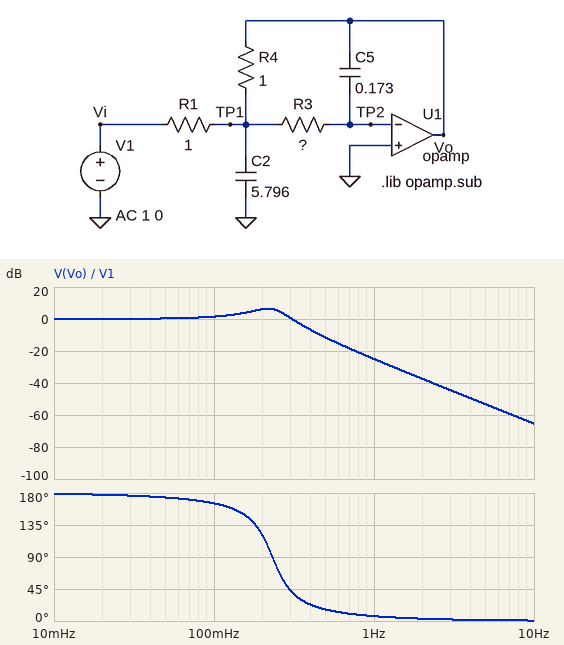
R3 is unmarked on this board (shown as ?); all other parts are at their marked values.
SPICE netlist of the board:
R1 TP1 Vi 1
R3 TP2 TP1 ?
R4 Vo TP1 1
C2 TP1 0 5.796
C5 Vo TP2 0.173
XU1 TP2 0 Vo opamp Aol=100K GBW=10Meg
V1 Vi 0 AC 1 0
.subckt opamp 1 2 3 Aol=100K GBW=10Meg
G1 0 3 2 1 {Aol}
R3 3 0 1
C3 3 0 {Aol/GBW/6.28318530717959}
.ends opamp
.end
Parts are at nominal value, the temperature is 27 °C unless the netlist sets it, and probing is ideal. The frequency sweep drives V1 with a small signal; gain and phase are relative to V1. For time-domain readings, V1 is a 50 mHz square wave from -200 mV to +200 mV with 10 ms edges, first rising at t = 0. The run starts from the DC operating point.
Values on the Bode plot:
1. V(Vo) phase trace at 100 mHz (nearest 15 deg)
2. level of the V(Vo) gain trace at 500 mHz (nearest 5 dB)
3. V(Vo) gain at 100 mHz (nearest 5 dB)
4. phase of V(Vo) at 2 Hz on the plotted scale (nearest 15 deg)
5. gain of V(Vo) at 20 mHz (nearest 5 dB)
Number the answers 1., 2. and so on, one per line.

1. 165 deg
2. -10 dB
3. 0 dB
4. 0 deg
5. 0 dB
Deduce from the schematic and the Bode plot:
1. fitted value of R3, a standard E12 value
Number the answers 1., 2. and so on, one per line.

1. 0.47 Ω
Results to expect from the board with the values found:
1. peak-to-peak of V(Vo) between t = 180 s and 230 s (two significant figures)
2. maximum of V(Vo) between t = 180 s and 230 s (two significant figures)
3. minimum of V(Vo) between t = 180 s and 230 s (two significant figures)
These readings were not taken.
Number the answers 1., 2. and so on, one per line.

1. 760 mV
2. 380 mV
3. -380 mV
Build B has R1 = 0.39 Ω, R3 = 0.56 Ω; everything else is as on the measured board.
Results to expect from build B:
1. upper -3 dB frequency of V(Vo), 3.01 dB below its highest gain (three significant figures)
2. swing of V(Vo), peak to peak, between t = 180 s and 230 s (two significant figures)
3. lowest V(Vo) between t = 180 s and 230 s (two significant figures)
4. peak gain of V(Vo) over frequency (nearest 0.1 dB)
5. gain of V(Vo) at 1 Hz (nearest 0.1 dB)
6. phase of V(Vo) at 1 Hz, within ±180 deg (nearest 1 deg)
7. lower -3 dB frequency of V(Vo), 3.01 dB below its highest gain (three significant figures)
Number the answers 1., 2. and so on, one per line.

1. 252 mHz
2. 1.7 V
3. -830 mV
4. 11.9 dB
5. -18.4 dB
6. 9 deg
7. 71.0 mHz
